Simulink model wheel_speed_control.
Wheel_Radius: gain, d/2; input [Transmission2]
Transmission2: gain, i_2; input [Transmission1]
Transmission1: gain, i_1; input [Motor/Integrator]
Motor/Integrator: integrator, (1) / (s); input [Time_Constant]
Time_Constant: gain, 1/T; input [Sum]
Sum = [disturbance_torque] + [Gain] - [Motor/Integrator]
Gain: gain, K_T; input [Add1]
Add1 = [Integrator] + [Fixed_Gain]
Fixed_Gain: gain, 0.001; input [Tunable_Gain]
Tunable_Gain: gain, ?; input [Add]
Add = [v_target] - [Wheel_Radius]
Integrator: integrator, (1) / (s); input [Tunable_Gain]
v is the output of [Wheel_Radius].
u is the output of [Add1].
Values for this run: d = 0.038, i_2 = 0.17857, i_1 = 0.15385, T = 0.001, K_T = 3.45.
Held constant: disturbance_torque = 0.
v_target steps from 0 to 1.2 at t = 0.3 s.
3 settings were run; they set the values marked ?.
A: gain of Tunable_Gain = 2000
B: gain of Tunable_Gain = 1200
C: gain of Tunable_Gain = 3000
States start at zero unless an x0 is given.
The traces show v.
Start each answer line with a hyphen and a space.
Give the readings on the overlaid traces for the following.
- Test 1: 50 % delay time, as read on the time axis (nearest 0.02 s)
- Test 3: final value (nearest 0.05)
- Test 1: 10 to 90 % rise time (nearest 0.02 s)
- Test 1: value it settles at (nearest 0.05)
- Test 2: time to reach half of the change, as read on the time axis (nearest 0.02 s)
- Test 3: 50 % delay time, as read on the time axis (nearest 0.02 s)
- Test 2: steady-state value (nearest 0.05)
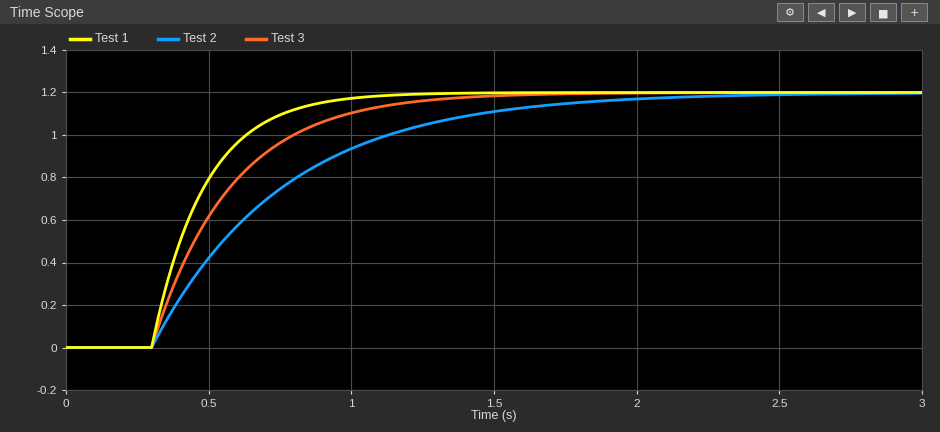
- 0.42 s
- 1.20
- 0.40 s
- 1.20
- 0.62 s
- 0.50 s
- 1.20
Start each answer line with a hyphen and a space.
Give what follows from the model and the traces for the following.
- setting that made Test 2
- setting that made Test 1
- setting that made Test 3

- B
- C
- A
